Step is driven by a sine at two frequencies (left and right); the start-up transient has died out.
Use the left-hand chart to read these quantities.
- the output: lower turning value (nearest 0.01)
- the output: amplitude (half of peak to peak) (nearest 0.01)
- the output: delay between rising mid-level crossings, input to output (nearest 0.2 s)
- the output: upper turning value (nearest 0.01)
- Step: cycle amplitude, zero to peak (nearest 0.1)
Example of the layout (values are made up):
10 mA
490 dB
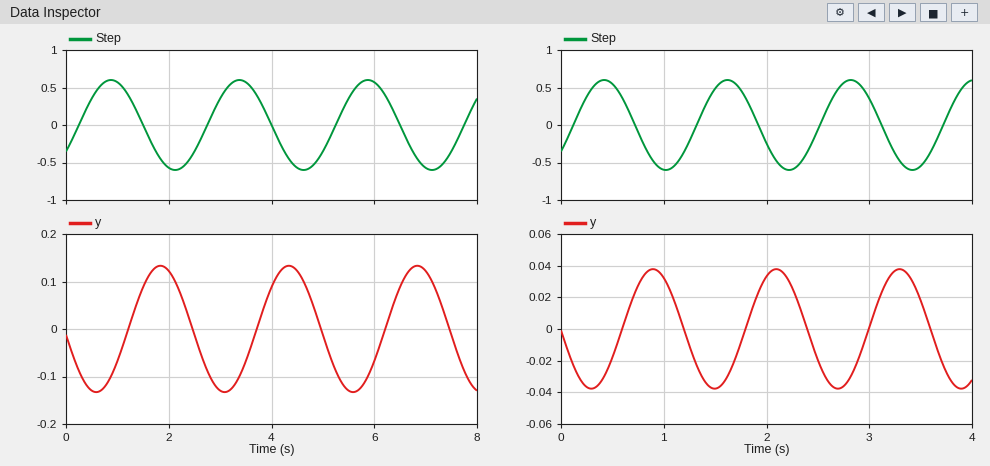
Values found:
-0.13
0.13
1.0 s
0.13
0.6
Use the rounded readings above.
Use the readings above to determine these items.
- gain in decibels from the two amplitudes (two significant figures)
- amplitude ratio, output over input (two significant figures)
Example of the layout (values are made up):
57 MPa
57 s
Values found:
-13 dB
0.22
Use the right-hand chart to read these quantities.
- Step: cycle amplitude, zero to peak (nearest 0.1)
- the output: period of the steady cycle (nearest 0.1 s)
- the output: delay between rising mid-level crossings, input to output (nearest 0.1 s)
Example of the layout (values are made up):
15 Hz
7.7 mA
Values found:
0.6
1.2 s
0.5 s
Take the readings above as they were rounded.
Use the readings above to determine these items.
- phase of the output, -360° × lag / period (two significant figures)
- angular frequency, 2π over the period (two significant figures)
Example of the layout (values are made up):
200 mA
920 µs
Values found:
-150°
5.2 rad/s
